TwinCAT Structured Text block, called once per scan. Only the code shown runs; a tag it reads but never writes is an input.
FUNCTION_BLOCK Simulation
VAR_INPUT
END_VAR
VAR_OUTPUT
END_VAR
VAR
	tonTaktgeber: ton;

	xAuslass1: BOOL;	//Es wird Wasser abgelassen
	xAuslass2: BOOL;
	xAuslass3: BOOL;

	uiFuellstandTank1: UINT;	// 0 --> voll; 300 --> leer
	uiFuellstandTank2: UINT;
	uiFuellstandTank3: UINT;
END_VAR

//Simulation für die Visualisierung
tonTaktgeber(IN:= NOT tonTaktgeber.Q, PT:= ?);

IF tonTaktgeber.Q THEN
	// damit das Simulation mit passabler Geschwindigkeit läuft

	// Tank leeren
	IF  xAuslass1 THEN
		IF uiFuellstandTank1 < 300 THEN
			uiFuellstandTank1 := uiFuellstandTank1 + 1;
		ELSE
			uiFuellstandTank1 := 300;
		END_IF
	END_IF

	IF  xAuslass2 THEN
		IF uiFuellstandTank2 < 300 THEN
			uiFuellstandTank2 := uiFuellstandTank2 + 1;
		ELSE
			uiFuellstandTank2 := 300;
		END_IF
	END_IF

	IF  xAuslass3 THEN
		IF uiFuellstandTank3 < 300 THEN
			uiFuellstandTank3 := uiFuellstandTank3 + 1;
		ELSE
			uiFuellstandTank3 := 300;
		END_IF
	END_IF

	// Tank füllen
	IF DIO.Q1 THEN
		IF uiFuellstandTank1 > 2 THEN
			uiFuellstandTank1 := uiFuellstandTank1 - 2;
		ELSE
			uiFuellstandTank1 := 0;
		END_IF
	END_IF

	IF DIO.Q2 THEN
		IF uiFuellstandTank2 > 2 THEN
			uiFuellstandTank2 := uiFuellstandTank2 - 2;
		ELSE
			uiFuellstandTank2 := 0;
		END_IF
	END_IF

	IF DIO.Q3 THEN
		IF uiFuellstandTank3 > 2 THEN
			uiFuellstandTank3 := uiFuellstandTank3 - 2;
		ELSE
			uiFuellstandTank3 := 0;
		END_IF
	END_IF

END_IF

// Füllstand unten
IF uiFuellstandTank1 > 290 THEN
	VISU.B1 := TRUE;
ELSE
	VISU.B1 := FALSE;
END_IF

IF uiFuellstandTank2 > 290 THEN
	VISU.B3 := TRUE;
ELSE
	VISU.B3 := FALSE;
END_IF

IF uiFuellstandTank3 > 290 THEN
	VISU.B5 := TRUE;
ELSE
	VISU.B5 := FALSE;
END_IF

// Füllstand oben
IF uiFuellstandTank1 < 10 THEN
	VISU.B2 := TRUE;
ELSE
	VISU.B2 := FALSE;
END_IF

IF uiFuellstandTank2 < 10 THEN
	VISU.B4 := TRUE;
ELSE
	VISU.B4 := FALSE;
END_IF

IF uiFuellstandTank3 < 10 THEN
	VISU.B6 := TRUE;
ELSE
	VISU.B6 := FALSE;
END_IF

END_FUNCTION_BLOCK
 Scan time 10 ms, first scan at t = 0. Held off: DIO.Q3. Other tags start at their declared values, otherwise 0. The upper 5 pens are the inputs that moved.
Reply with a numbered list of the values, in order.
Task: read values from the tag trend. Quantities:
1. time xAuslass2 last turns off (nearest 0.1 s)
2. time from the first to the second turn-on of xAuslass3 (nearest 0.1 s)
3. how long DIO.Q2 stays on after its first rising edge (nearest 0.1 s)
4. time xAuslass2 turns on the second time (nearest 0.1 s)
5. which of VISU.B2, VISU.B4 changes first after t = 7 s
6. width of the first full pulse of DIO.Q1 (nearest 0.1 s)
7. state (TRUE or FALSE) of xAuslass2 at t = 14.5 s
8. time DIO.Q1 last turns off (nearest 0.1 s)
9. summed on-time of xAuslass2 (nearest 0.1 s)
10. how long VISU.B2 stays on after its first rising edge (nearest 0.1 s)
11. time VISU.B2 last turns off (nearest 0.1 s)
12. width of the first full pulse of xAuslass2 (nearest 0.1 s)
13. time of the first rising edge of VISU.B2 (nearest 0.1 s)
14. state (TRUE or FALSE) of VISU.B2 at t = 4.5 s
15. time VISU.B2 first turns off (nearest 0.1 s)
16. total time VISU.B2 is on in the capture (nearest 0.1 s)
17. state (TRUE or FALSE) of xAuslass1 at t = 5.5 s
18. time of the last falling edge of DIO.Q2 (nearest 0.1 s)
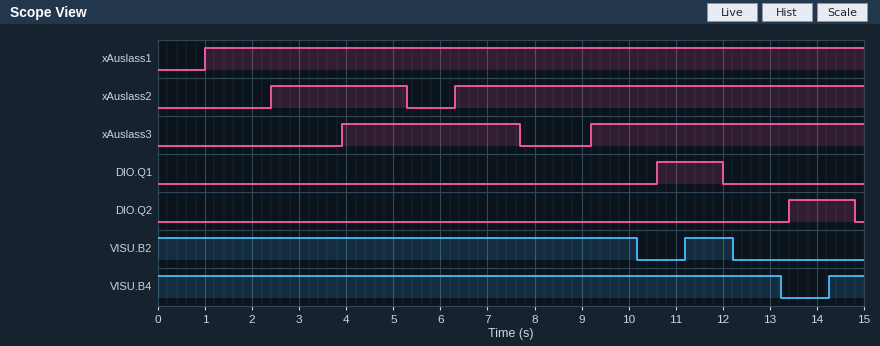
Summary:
1. 5.3 s
2. 5.3 s
3. 1.4 s
4. 6.3 s
5. VISU.B2
6. 1.4 s
7. TRUE
8. 12.0 s
9. 11.6 s
10. 1.0 s
11. 12.2 s
12. 2.9 s
13. 11.2 s
14. TRUE
15. 10.2 s
16. 11.2 s
17. TRUE
18. 14.8 s
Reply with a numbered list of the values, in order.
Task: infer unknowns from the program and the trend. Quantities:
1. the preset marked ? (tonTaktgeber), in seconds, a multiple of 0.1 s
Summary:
1. 1.0 s
